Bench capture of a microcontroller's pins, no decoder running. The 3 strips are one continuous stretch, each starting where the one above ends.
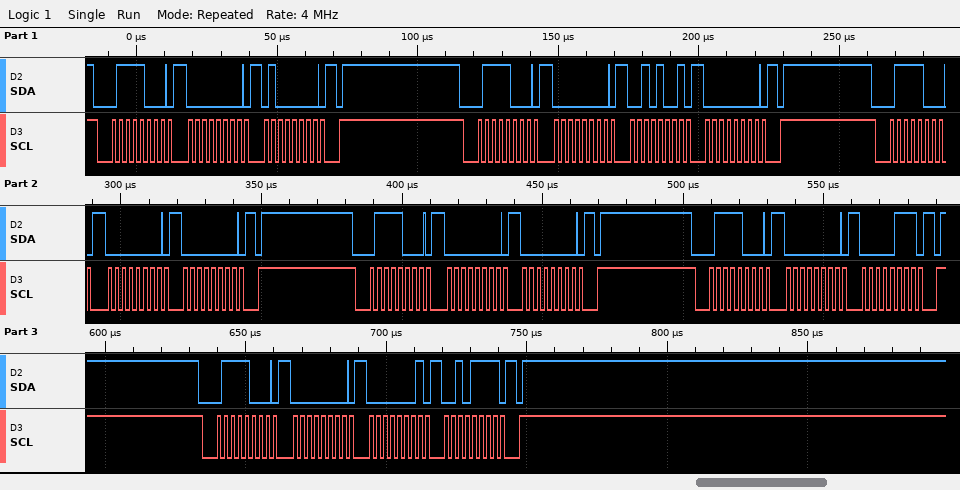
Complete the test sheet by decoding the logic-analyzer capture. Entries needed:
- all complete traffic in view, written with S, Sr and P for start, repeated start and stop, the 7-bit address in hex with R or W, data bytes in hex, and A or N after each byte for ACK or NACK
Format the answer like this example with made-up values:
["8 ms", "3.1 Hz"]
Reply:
["S 3CW A 00 A 40 A P S 3CW A 00 A 29 A 00 A P S 3CW A 00 A 00 A P S 3CW A 00 A 00 A P S 3CW A 00 A 07 A P S 3CW A 00 A 01 A 2F A P"]
